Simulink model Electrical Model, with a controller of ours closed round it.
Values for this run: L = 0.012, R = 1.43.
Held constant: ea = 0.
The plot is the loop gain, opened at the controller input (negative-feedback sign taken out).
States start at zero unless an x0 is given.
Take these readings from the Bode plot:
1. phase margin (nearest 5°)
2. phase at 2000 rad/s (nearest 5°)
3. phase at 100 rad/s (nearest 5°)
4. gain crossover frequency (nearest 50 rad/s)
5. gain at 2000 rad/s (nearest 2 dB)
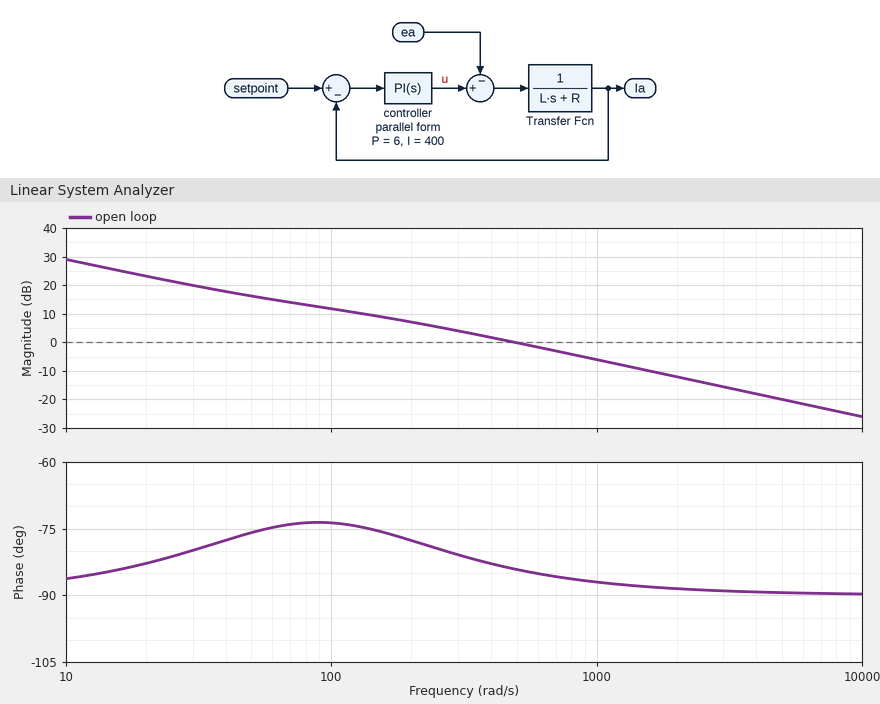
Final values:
95°
-90°
-75°
500 rad/s
-12 dB
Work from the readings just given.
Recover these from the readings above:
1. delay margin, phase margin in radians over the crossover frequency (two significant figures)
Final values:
0.0033 s
